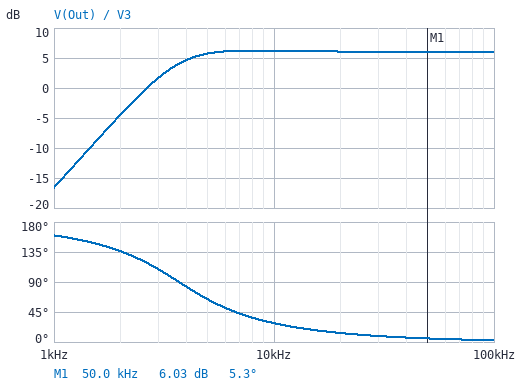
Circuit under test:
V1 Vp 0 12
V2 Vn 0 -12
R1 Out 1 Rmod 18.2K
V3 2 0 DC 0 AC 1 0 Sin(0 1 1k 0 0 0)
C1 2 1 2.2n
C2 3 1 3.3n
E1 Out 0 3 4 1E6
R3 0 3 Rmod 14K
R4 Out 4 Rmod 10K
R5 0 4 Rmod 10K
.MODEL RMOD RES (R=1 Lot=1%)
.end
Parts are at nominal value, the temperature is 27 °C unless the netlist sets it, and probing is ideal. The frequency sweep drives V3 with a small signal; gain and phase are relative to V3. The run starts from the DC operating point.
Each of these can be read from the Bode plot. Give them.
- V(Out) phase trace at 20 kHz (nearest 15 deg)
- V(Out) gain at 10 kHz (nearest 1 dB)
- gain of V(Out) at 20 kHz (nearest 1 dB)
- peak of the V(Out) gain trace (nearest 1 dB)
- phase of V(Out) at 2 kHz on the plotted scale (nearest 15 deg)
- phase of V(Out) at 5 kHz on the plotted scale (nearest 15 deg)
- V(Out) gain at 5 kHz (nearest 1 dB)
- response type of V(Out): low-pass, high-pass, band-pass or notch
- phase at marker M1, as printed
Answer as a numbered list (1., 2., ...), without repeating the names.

1. 15 deg
2. 6 dB
3. 6 dB
4. 6 dB
5. 135 deg
6. 60 deg
7. 6 dB
8. high-pass
9. 5.3 deg
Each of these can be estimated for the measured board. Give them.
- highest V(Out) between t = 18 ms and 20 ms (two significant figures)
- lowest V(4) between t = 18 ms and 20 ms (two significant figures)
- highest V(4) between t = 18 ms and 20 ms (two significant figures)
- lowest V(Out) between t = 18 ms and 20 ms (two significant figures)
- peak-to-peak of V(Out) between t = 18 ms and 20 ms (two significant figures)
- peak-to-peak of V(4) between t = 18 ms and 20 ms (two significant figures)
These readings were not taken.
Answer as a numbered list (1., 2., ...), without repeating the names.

1. 150 mV
2. -74 mV
3. 74 mV
4. -150 mV
5. 300 mV
6. 150 mV
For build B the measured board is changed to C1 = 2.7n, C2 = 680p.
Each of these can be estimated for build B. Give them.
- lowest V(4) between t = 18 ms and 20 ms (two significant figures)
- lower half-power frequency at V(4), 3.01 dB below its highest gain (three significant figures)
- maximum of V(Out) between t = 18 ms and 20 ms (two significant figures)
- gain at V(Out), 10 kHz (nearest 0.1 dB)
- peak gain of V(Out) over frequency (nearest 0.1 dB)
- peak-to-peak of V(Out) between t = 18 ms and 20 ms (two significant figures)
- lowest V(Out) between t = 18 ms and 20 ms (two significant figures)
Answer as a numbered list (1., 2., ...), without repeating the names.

1. -18 mV
2. 14.8 kHz
3. 36 mV
4. 0.8 dB
5. 6.0 dB
6. 71 mV
7. -36 mV
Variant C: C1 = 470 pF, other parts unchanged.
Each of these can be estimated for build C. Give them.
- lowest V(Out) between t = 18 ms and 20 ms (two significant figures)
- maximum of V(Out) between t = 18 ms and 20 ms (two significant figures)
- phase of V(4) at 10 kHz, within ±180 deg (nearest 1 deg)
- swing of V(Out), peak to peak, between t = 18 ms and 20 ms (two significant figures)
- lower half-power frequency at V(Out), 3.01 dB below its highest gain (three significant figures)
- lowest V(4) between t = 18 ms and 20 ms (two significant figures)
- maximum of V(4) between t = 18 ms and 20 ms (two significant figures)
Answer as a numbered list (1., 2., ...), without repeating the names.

1. -31 mV
2. 31 mV
3. 68 deg
4. 63 mV
5. 7.03 kHz
6. -16 mV
7. 16 mV
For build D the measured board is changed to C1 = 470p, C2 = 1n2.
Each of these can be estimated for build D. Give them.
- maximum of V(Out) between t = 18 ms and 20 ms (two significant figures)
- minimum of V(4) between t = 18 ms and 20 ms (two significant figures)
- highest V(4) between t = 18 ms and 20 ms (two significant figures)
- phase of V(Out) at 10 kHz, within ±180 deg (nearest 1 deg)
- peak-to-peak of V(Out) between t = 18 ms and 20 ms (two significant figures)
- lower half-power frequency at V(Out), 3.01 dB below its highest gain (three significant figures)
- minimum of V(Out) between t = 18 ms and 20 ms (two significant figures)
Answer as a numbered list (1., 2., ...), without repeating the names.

1. 11 mV
2. -5.7 mV
3. 5.7 mV
4. 117 deg
5. 23 mV
6. 11.7 kHz
7. -11 mV
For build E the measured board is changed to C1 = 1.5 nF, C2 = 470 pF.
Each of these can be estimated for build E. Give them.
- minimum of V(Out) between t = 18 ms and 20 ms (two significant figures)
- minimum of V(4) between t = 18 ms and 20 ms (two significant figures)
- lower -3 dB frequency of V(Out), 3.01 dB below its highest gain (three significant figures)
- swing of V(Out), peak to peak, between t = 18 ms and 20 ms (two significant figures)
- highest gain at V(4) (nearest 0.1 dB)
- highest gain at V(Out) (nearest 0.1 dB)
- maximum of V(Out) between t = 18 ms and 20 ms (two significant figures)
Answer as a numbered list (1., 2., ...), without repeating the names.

1. -14 mV
2. -7.0 mV
3. 20.9 kHz
4. 28 mV
5. 0 dB
6. 6.0 dB
7. 14 mV
